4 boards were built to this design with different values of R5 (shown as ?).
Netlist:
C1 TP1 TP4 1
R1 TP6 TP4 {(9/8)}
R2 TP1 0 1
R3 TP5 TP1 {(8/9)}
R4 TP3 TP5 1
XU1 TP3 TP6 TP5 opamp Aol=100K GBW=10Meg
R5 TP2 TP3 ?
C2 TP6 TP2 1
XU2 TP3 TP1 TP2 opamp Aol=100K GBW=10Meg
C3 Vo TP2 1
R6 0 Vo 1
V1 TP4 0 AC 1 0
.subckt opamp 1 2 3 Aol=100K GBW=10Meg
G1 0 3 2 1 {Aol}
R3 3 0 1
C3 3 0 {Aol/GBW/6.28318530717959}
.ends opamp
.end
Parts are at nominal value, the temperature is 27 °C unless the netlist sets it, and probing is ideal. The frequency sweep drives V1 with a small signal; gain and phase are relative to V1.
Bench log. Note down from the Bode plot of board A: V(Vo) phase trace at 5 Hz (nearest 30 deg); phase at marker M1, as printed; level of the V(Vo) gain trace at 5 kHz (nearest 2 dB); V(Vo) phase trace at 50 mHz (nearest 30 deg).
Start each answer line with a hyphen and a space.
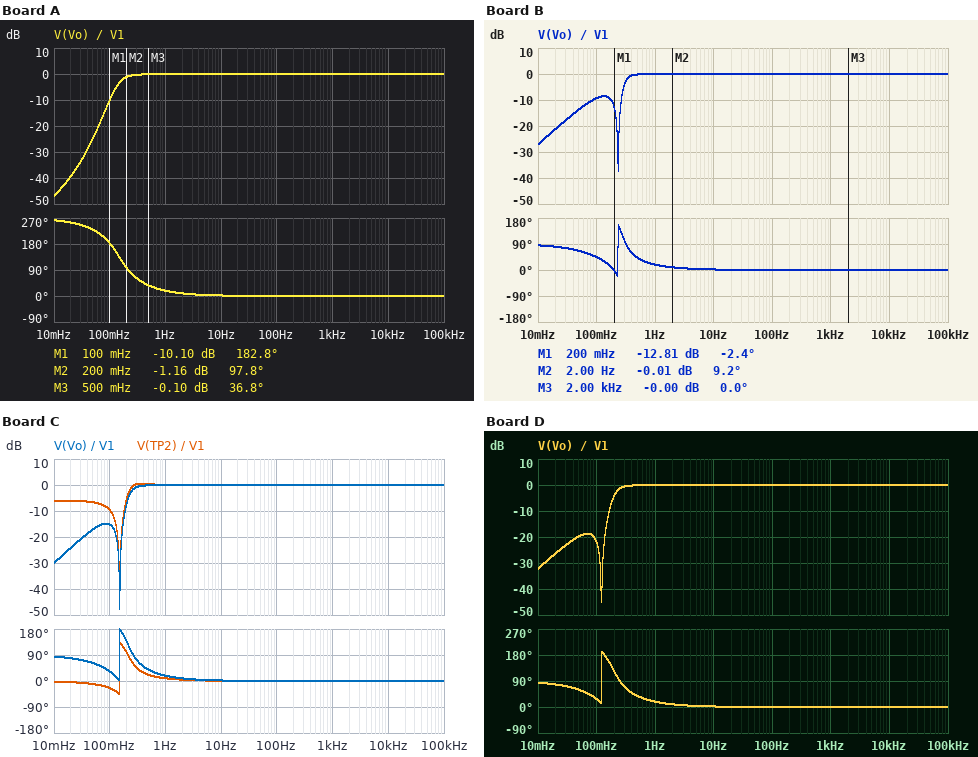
- 0 deg
- 182.8 deg
- 0 dB
- 240 deg
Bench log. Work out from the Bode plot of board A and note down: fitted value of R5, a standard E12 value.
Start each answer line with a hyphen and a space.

- 1.2 Ω
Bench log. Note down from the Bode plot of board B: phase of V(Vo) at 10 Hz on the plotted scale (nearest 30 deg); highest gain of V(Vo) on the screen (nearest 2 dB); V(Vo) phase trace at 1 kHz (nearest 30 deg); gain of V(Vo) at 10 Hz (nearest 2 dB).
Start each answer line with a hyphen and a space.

- 0 deg
- 0 dB
- 0 deg
- 0 dB
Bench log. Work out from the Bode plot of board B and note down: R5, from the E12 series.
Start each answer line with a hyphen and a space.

- 0.33 Ω
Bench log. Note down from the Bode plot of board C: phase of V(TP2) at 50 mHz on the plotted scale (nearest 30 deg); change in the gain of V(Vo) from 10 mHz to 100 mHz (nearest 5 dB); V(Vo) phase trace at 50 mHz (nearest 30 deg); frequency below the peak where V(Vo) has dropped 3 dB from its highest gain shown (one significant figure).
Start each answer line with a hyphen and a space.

- 0 deg
- 15 dB
- 60 deg
- 200 mHz
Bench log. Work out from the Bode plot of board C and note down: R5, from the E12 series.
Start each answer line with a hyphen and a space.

- 0.56 Ω
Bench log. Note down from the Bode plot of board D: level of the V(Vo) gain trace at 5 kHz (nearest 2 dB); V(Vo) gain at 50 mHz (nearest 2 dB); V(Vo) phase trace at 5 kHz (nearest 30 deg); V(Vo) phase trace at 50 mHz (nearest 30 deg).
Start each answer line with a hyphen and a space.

- 0 dB
- -20 dB
- 0 deg
- 60 deg
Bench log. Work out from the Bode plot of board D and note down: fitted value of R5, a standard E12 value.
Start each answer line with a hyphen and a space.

- 0.68 Ω
